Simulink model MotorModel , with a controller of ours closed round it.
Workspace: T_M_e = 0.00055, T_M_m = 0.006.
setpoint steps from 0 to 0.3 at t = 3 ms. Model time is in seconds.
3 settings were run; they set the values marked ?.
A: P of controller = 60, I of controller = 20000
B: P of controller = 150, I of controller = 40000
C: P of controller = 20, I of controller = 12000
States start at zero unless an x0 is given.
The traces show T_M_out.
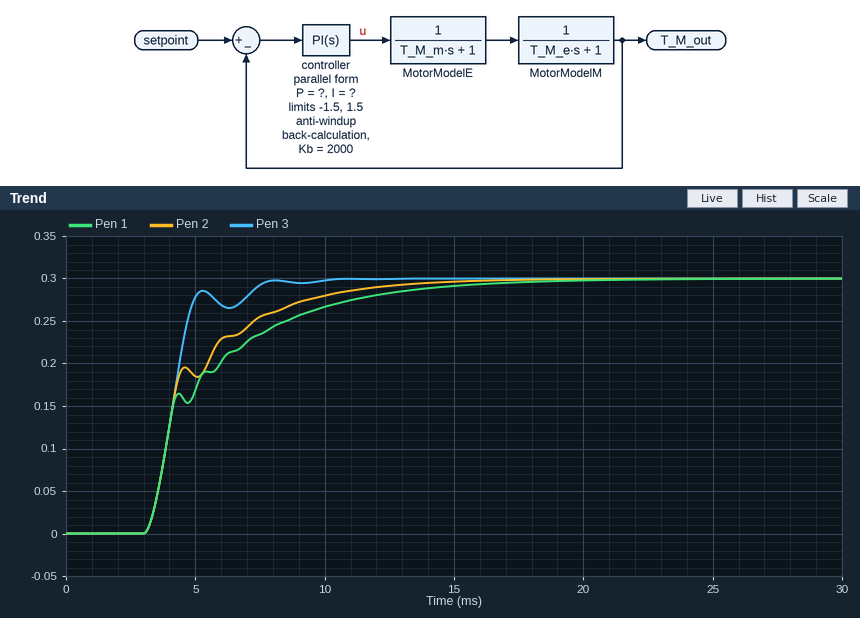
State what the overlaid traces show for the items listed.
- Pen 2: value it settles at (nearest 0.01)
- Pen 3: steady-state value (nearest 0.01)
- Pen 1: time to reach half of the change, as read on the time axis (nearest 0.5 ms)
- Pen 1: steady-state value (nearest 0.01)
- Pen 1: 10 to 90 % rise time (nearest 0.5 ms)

0.30
0.30
4.0 ms
0.30
7.0 ms
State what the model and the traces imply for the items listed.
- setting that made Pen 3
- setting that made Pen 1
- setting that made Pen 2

C
B
A
